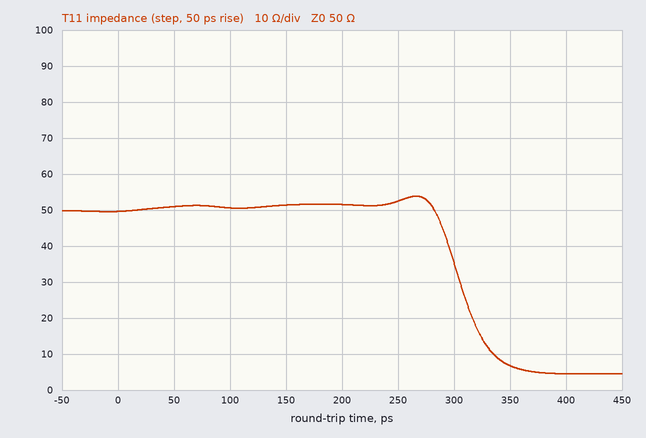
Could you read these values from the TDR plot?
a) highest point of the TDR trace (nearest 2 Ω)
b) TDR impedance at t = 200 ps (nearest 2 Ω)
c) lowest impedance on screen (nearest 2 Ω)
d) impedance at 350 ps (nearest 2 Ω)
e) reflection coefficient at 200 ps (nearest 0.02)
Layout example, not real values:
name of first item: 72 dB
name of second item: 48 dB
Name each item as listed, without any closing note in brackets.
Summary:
highest point of the TDR trace: 54 Ω
TDR impedance at t = 200 ps: 52 Ω
lowest impedance on screen: 4 Ω
impedance at 350 ps: 6 Ω
reflection coefficient at 200 ps: +0.02
